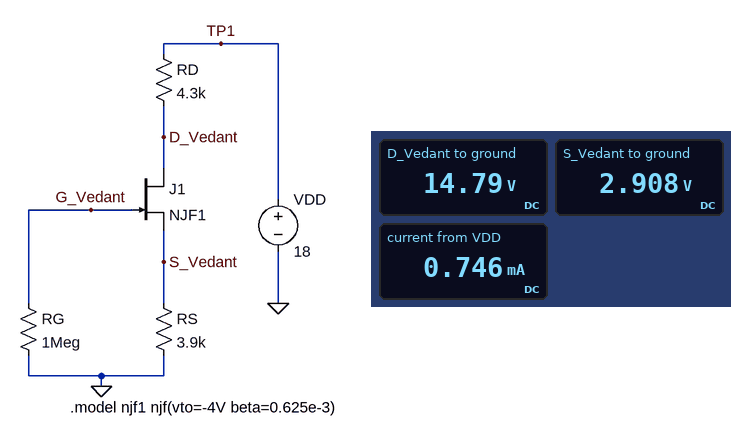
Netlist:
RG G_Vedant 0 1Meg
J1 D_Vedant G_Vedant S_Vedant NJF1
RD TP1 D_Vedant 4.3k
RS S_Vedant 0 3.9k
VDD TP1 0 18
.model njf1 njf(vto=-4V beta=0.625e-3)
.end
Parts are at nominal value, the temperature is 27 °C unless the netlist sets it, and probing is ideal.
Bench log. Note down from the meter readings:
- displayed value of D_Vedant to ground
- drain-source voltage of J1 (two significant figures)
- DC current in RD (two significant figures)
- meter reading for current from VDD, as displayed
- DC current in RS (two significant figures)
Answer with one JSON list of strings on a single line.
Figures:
["14.79 V", "12 V", "750 µA", "0.746 mA", "750 µA"]
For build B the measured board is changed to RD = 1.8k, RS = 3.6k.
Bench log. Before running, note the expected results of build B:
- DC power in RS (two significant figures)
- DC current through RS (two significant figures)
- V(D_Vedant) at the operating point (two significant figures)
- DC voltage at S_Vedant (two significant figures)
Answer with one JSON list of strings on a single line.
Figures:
["2.3 mW", "800 µA", "17 V", "2.9 V"]
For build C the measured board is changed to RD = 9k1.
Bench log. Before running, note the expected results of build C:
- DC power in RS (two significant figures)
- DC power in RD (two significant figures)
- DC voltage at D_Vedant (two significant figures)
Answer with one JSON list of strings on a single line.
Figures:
["2.2 mW", "5.1 mW", "11 V"]
